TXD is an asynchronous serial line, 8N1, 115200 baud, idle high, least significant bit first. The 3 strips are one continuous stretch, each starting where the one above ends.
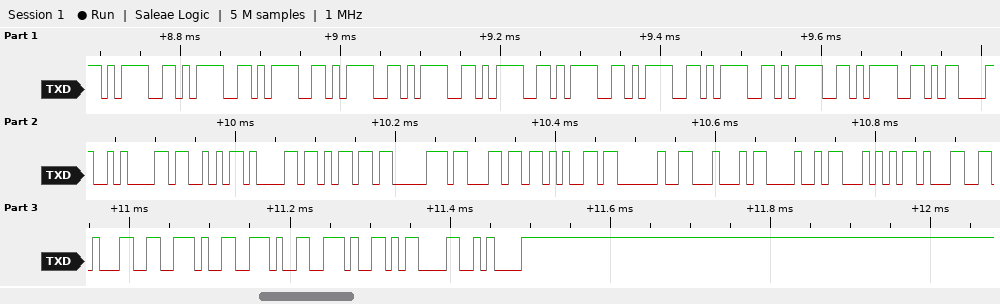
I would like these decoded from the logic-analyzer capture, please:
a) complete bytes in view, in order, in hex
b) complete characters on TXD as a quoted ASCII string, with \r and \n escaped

3D 3D 3D 3D 3D 3D 3D 3D 3D 3D 3D 0D 0A 53 61 6D 70 6C 65 20 44 48 54 31 31 2E 2E 2E 0D 0A
"===========\r\nSample DHT11...\r\n"
